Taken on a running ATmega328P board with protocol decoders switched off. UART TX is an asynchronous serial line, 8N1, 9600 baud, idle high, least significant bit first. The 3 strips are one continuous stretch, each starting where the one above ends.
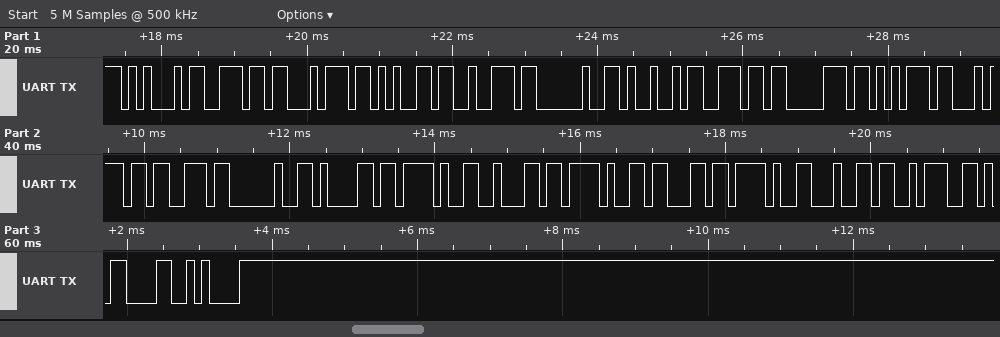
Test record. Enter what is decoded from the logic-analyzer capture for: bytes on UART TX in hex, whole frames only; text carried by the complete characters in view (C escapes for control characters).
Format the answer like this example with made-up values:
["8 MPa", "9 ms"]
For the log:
["45 6E 74 65 72 20 49 6E 70 75 74 73 20 61 2F 62 2F 63 2F 64 3A 0D 0A", "\"Enter Inputs a/b/c/d:\\r\\n\""]
